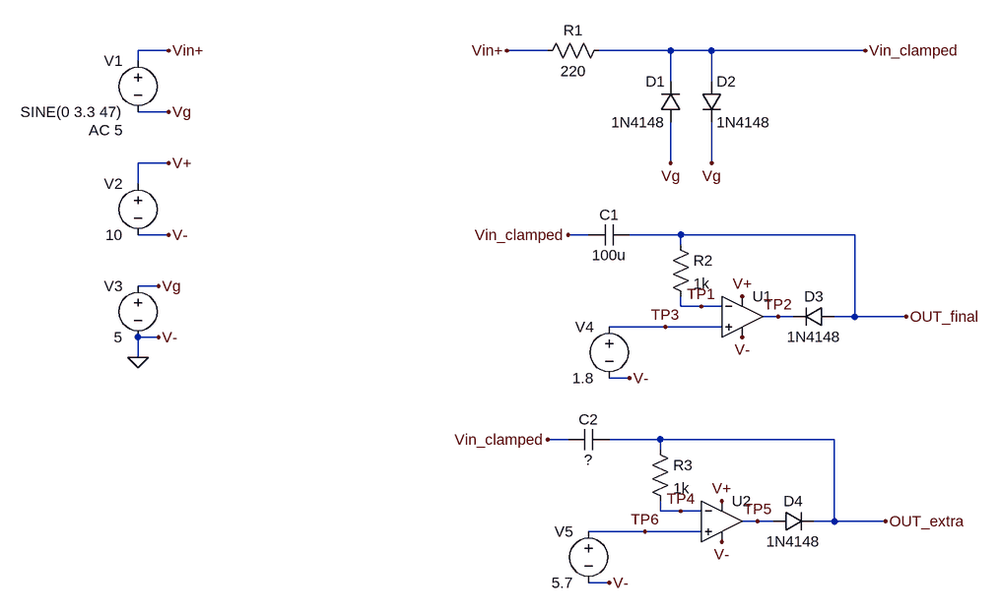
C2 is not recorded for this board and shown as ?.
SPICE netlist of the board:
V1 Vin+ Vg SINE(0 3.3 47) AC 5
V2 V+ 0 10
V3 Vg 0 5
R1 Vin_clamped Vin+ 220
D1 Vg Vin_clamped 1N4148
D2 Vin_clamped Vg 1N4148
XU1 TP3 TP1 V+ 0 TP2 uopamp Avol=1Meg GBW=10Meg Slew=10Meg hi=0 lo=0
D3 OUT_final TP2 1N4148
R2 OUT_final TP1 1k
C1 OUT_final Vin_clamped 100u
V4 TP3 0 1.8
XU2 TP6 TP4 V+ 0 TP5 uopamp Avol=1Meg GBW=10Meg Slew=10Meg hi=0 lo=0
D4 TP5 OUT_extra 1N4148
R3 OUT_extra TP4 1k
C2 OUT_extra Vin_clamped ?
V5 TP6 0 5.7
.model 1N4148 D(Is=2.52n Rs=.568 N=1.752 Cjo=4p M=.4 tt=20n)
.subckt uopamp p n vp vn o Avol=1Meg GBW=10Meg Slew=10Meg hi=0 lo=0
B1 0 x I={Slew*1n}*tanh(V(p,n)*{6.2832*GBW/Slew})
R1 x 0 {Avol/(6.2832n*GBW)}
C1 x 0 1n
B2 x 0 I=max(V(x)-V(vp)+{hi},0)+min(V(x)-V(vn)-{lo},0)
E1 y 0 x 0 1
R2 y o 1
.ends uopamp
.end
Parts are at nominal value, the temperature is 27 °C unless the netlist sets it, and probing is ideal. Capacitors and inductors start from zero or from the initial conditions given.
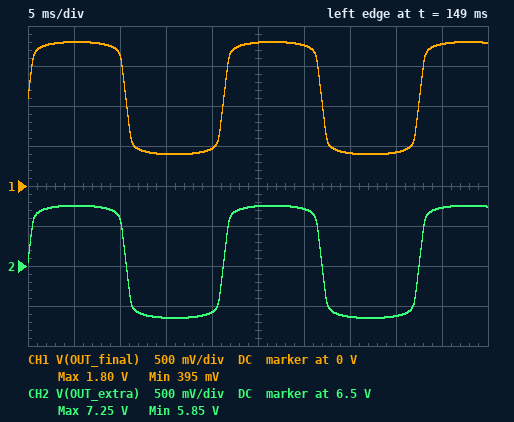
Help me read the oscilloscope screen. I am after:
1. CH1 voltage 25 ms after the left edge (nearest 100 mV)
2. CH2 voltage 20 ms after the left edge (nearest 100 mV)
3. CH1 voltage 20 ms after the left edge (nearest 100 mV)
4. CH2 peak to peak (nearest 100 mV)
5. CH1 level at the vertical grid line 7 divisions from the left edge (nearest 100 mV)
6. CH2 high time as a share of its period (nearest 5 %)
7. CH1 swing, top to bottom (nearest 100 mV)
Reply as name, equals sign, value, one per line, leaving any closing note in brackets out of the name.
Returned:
CH1 voltage 25 ms after the left edge = 1.8 V
CH2 voltage 20 ms after the left edge = 5.9 V
CH1 voltage 20 ms after the left edge = 500 mV
CH2 peak to peak = 1.4 V
CH1 level at the vertical grid line 7 divisions from the left edge = 400 mV
CH2 high time as a share of its period = 50 %
CH1 swing, top to bottom = 1.4 V
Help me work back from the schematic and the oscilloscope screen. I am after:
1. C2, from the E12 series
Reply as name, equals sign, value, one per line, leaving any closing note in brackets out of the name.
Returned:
C2, from the E12 series = 150 µF
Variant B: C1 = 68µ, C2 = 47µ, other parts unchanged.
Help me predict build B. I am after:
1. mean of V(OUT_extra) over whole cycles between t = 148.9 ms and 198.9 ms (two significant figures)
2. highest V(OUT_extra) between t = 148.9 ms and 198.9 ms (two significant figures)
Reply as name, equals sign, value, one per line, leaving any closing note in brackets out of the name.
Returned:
mean of V(OUT_extra) over whole cycles between t = 148.9 ms and 198.9 ms = 7.0 V
highest V(OUT_extra) between t = 148.9 ms and 198.9 ms = 7.7 V
